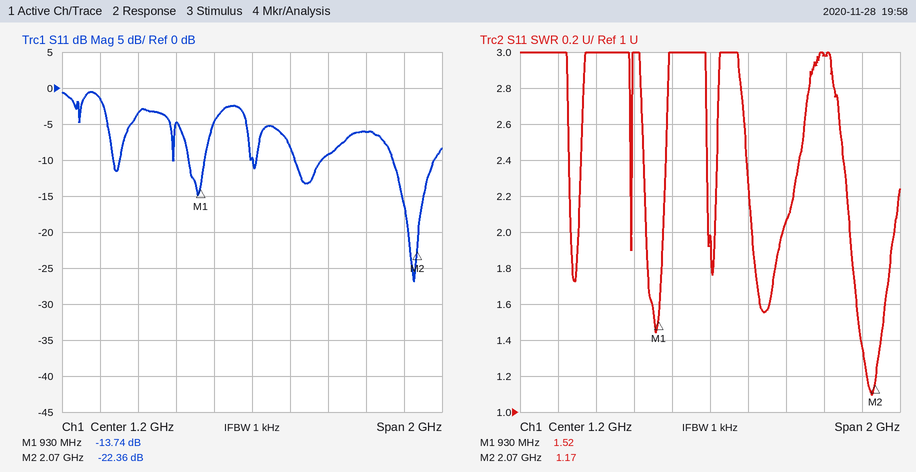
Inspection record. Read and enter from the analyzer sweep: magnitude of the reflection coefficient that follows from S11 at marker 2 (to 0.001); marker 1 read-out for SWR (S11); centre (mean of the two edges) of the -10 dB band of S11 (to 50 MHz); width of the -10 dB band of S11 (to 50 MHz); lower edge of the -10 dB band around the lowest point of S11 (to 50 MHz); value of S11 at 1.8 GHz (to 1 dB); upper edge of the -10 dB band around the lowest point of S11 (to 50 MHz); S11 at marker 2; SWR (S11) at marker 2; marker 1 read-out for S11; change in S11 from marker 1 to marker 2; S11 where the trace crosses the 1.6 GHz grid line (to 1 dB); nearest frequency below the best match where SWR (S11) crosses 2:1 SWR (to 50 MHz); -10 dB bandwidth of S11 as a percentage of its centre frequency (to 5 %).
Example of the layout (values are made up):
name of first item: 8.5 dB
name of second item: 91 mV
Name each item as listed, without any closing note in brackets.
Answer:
magnitude of the reflection coefficient that follows from S11 at marker 2: 0.076
marker 1 read-out for SWR: 1.52
centre (mean of the two edges) of the -10 dB band of S11: 2.05 GHz
width of the -10 dB band of S11: 200 MHz
lower edge of the -10 dB band around the lowest point of S11: 1.95 GHz
value of S11 at 1.8 GHz: -6 dB
upper edge of the -10 dB band around the lowest point of S11: 2.15 GHz
S11 at marker 2: -22.36 dB
SWR (S11) at marker 2: 1.17
marker 1 read-out for S11: -13.74 dB
change in S11 from marker 1 to marker 2: -8.62 dB
S11 where the trace crosses the 1.6 GHz grid line: -9 dB
nearest frequency below the best match where SWR (S11) crosses 2:1 SWR: 1.95 GHz
-10 dB bandwidth of S11 as a percentage of its centre frequency: 10 %
